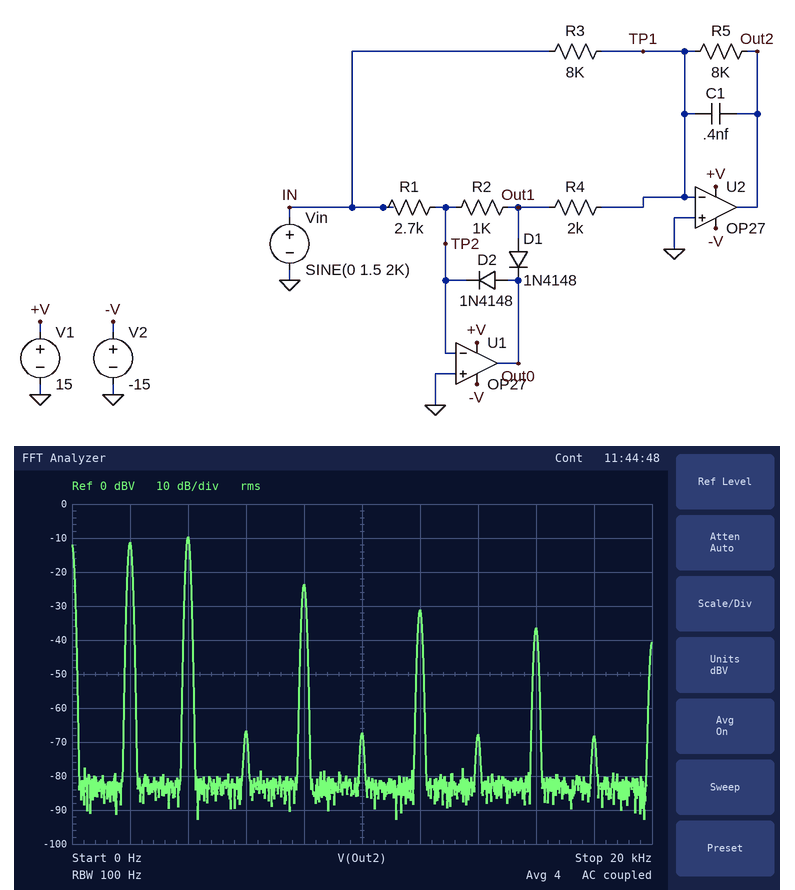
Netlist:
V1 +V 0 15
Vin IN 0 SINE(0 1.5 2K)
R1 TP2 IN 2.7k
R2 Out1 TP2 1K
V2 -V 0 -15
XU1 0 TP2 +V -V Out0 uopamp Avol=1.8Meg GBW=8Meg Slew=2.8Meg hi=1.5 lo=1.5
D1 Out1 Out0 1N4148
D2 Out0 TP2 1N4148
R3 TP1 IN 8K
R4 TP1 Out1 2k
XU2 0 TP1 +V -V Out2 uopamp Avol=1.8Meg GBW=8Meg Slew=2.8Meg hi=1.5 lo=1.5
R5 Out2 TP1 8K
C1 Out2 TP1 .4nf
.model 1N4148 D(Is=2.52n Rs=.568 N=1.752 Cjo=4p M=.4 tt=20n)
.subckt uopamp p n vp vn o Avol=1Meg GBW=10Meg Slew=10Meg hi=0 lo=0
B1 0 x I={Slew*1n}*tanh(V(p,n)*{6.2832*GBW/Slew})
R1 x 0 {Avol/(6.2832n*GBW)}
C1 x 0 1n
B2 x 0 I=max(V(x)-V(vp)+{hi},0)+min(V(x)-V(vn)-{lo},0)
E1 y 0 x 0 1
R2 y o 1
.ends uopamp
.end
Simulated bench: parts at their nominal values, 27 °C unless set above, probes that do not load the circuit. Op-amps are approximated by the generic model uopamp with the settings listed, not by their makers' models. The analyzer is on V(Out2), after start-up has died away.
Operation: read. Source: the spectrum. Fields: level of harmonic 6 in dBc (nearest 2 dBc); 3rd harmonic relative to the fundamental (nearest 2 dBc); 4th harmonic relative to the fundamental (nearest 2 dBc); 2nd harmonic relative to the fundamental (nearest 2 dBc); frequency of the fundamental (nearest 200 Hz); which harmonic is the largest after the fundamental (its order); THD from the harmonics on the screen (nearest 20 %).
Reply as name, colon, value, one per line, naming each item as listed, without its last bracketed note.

level of harmonic 6 in dBc: -20 dBc
3rd harmonic relative to the fundamental: -56 dBc
4th harmonic relative to the fundamental: -12 dBc
2nd harmonic relative to the fundamental: 2 dBc
frequency of the fundamental: 2.0 kHz
which harmonic is the largest after the fundamental: 2
THD from the harmonics on the screen: 120 %
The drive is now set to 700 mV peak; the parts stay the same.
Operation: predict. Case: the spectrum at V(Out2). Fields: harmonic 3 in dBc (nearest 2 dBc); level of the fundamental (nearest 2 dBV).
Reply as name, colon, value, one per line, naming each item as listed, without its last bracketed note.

harmonic 3 in dBc: -50 dBc
level of the fundamental: -18 dBV
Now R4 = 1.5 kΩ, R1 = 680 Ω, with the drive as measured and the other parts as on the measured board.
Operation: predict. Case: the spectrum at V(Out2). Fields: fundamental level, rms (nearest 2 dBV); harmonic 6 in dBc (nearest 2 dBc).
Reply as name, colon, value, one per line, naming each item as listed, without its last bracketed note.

fundamental level, rms: 10 dBV
harmonic 6 in dBc: -26 dBc
